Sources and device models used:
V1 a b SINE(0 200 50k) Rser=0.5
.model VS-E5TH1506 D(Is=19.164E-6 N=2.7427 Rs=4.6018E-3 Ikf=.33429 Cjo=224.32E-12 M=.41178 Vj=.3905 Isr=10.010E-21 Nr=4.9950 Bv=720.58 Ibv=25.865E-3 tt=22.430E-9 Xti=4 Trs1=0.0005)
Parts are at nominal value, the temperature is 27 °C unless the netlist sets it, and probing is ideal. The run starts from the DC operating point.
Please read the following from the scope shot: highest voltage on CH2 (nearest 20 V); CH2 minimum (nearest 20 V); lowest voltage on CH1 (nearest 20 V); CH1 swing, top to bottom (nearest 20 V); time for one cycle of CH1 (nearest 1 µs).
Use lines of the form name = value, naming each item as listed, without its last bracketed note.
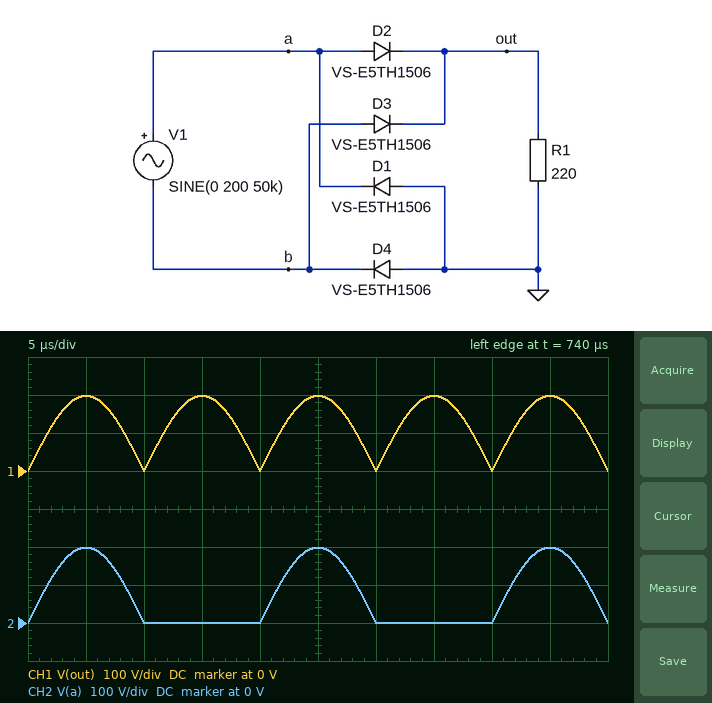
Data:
highest voltage on CH2 = 200 V
CH2 minimum = 0 V
lowest voltage on CH1 = 0 V
CH1 swing, top to bottom = 200 V
time for one cycle of CH1 = 10 µs
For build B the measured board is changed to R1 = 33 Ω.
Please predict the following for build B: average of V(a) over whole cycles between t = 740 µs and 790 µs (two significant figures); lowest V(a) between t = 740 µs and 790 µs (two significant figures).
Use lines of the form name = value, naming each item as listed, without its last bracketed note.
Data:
average of V(a) over whole cycles between t = 740 µs and 790 µs = 62 V
lowest V(a) between t = 740 µs and 790 µs = -1.1 V
